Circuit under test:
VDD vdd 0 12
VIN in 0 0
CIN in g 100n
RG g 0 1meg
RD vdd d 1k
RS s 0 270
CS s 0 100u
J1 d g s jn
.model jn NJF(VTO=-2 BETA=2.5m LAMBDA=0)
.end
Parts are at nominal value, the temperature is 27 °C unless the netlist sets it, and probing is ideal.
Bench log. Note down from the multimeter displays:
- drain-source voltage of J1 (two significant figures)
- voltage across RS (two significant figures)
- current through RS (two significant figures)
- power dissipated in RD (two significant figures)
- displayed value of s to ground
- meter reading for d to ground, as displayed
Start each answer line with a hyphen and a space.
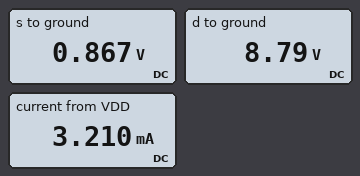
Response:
- 7.9 V
- 870 mV
- 3.2 mA
- 10 mW
- 0.867 V
- 8.79 V
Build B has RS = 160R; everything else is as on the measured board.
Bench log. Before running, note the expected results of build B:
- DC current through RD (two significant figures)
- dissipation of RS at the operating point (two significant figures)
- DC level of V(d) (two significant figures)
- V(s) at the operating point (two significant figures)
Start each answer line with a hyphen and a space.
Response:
- 4.3 mA
- 3.0 mW
- 7.7 V
- 690 mV
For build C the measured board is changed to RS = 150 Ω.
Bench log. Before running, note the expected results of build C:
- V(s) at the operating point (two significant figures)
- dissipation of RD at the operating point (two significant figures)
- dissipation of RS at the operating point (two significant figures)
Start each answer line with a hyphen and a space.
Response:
- 670 mV
- 20 mW
- 3.0 mW
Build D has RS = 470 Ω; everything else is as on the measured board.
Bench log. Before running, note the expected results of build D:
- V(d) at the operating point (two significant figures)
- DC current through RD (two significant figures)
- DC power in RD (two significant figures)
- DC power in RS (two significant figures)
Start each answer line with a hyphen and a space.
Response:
- 9.8 V
- 2.2 mA
- 5.0 mW
- 2.4 mW
